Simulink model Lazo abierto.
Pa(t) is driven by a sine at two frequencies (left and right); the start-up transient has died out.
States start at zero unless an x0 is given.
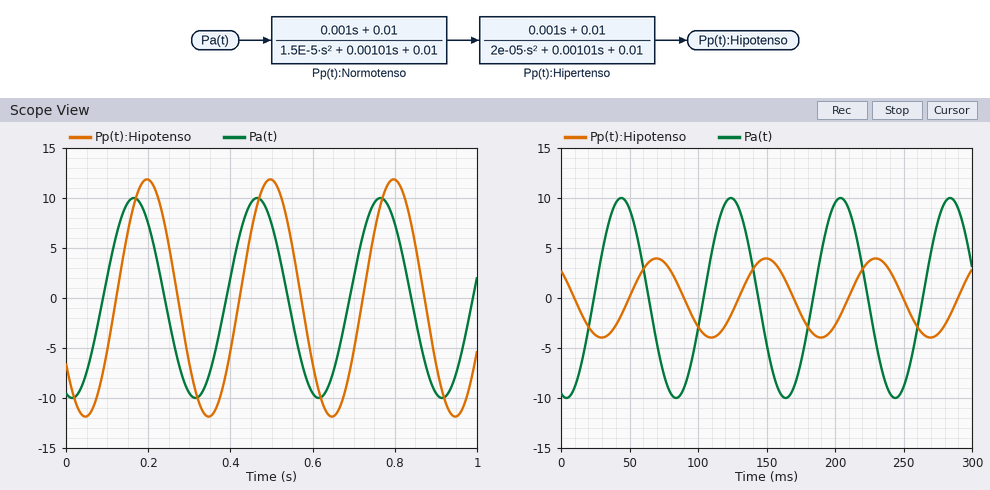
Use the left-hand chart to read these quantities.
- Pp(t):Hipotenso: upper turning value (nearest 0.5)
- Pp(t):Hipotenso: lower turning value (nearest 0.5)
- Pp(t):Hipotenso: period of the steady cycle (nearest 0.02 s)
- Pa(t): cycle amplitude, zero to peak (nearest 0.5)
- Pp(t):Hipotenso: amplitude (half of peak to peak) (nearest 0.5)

12.0
-12.0
0.30 s
10.0
12.0
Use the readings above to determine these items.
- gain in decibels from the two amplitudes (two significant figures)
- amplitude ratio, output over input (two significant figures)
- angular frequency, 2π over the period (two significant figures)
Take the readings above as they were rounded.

1.6 dB
1.2
21 rad/s
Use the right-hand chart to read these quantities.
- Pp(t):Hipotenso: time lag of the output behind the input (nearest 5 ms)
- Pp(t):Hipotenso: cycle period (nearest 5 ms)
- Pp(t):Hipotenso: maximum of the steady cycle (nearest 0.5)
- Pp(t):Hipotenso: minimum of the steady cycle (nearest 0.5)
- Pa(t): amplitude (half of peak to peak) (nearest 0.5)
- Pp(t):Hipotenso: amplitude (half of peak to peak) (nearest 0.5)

25 ms
80 ms
4.0
-4.0
10.0
4.0
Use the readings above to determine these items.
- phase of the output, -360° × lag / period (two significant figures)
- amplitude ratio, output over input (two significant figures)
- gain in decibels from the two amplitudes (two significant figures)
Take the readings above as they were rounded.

-110°
0.40
-8.0 dB
